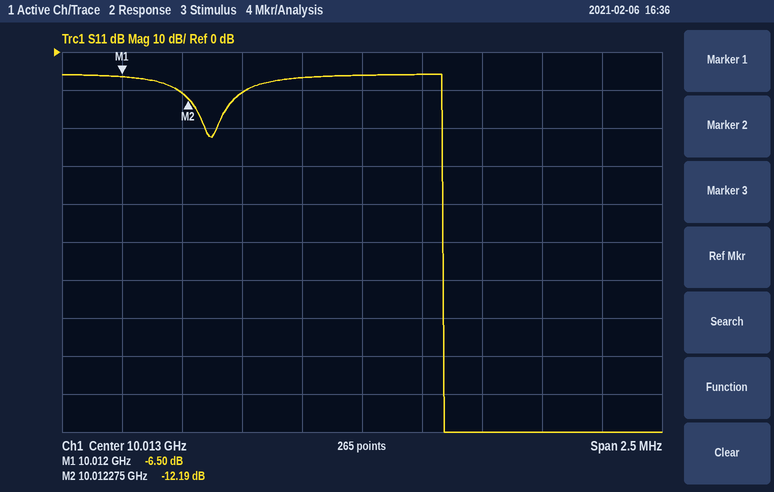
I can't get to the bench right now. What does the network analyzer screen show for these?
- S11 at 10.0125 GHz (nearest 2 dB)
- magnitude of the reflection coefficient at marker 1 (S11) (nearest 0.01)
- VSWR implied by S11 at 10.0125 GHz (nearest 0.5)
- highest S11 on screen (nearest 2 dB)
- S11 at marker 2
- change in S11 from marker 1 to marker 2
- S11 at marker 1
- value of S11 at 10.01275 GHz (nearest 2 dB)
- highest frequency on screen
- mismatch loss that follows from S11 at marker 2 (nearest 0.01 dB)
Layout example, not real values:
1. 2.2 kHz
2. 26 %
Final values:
1. -10 dB
2. 0.47
3. 2.0
4. -6 dB
5. -12.19 dB
6. -5.69 dB
7. -6.50 dB
8. -6 dB
9. 10.01425 GHz
10. 0.27 dB
